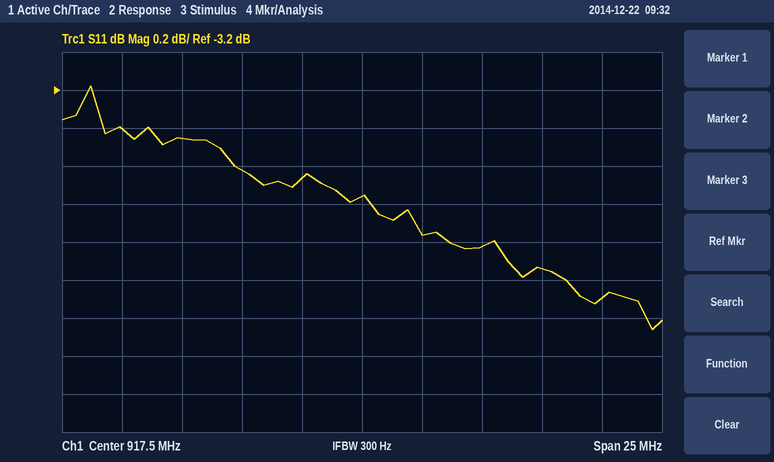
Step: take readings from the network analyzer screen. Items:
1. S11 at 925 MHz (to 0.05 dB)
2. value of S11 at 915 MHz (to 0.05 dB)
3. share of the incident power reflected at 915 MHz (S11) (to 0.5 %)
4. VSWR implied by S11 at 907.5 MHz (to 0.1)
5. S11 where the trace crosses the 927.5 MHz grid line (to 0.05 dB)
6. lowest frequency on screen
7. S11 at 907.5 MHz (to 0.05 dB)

-4.15 dB
-3.65 dB
43.0 %
5.2
-4.30 dB
905 MHz
-3.40 dB
